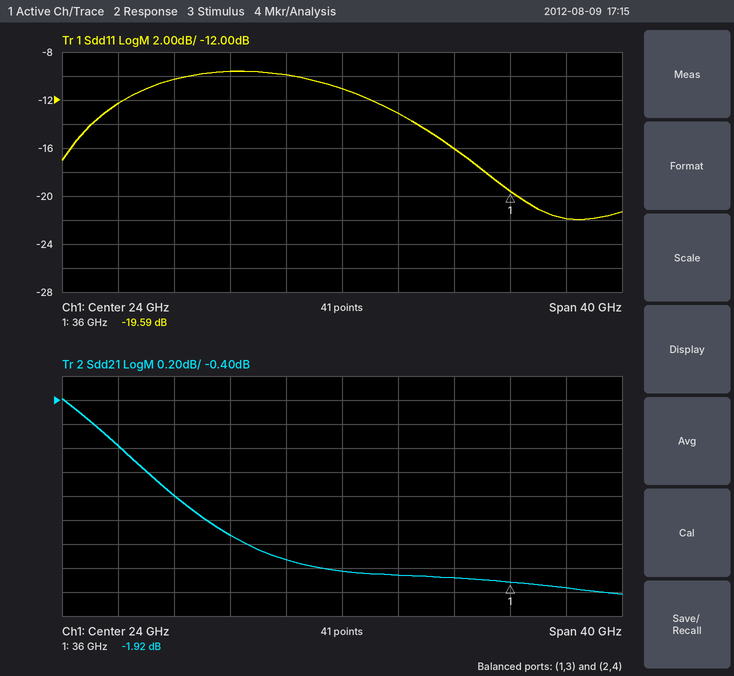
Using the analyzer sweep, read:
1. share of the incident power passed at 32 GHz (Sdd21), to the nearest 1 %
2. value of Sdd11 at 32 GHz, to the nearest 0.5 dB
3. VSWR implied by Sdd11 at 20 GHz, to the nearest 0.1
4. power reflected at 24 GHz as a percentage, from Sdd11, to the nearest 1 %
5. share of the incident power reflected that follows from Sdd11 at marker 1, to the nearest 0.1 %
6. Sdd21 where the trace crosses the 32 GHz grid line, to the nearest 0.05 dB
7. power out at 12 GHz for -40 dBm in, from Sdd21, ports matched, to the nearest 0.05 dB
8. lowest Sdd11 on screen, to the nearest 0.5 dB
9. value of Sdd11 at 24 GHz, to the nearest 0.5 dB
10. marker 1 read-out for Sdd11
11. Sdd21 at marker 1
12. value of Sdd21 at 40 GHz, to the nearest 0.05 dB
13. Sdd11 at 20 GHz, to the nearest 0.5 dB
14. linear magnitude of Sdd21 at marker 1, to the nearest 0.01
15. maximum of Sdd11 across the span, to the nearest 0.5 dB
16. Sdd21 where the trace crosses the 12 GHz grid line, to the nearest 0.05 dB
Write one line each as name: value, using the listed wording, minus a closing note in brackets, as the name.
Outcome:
share of the incident power passed at 32 GHz (Sdd21), to the nearest 1 %: 65 %
value of Sdd11 at 32 GHz, to the nearest 0.5 dB: -16.0 dB
VSWR implied by Sdd11 at 20 GHz, to the nearest 0.1: 1.9
power reflected at 24 GHz as a percentage, from Sdd11, to the nearest 1 %: 8 %
share of the incident power reflected that follows from Sdd11 at marker 1, to the nearest 0.1 %: 1.1 %
Sdd21 where the trace crosses the 32 GHz grid line, to the nearest 0.05 dB: -1.90 dB
power out at 12 GHz for -40 dBm in, from Sdd21, ports matched, to the nearest 0.05 dB: -41.20 dBm
lowest Sdd11 on screen, to the nearest 0.5 dB: -22.0 dB
value of Sdd11 at 24 GHz, to the nearest 0.5 dB: -11.0 dB
marker 1 read-out for Sdd11: -19.59 dB
Sdd21 at marker 1: -1.92 dB
value of Sdd21 at 40 GHz, to the nearest 0.05 dB: -1.95 dB
Sdd11 at 20 GHz, to the nearest 0.5 dB: -10.0 dB
linear magnitude of Sdd21 at marker 1, to the nearest 0.01: 0.80
maximum of Sdd11 across the span, to the nearest 0.5 dB: -9.5 dB
Sdd21 where the trace crosses the 12 GHz grid line, to the nearest 0.05 dB: -1.20 dB
